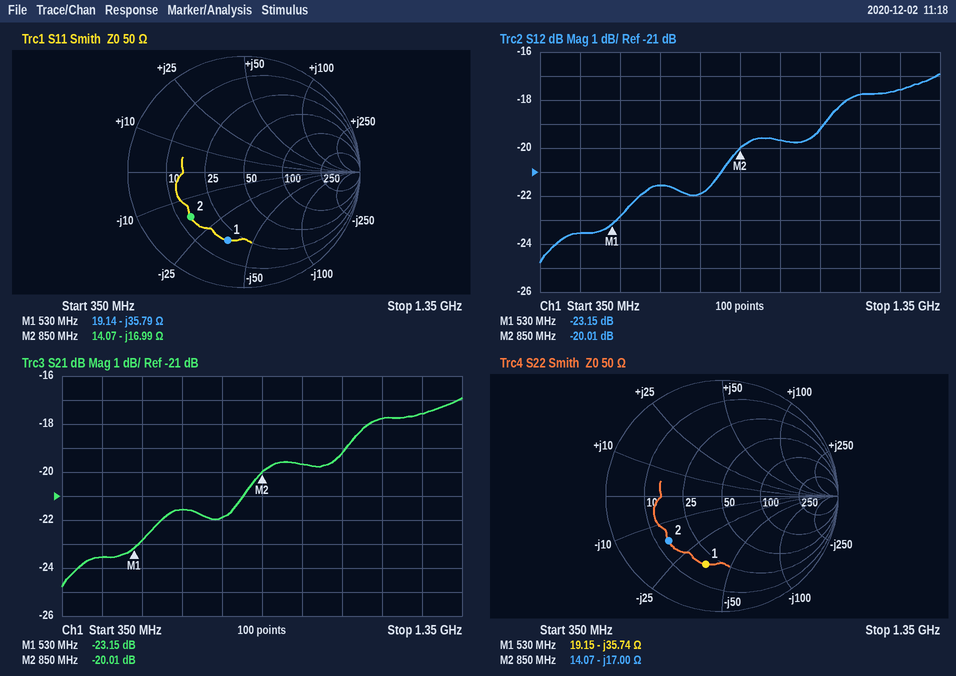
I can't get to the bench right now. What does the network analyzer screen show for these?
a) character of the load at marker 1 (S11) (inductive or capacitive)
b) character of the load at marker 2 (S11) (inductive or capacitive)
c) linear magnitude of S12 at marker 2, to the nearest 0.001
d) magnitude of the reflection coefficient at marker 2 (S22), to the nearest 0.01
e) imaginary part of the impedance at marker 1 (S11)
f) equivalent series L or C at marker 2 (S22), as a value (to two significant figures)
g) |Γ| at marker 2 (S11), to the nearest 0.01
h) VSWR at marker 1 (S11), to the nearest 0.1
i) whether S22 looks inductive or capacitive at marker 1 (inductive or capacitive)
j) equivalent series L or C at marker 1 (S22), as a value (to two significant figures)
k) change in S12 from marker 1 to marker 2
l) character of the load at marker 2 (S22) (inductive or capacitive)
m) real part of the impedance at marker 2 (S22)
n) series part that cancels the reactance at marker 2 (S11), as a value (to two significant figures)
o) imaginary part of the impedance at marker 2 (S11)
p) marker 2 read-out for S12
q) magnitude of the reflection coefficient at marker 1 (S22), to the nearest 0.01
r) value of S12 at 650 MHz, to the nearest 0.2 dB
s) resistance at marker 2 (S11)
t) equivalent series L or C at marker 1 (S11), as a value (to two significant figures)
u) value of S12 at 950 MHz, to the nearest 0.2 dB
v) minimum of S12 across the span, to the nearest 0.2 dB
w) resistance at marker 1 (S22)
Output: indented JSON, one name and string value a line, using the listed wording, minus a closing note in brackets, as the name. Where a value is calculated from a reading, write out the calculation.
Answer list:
{
  "character of the load at marker 1 (S11)": "capacitive",
  "character of the load at marker 2 (S11)": "capacitive",
  "linear magnitude of S12 at marker 2, to the nearest 0.001": "10^(-20.01/20) ≈ 0.100",
  "magnitude of the reflection coefficient at marker 2 (S22), to the nearest 0.01": "0.60",
  "imaginary part of the impedance at marker 1": "-35.79 Ω",
  "equivalent series L or C at marker 2 (S22), as a value": "C = 1/(2π × 850 MHz × 17 Ω) ≈ 11 pF",
  "|Γ| at marker 2 (S11), to the nearest 0.01": "0.60",
  "VSWR at marker 1 (S11), to the nearest 0.1": "4.1",
  "whether S22 looks inductive or capacitive at marker 1": "capacitive",
  "equivalent series L or C at marker 1 (S22), as a value": "C = 1/(2π × 530 MHz × 35.74 Ω) ≈ 8.4 pF",
  "change in S12 from marker 1 to marker 2": "-20.01 − (-23.15) = 3.14 dB",
  "character of the load at marker 2 (S22)": "capacitive",
  "real part of the impedance at marker 2": "14.07 Ω",
  "series part that cancels the reactance at marker 2 (S11), as a value": "L = 16.99 Ω/(2π × 850 MHz) ≈ 3.2 nH",
  "imaginary part of the impedance at marker 2": "-16.99 Ω",
  "marker 2 read-out for S12": "-20.01 dB",
  "magnitude of the reflection coefficient at marker 1 (S22), to the nearest 0.01": "0.61",
  "value of S12 at 650 MHz, to the nearest 0.2 dB": "-21.6 dB",
  "resistance at marker 2": "14.07 Ω",
  "equivalent series L or C at marker 1 (S11), as a value": "C = 1/(2π × 530 MHz × 35.79 Ω) ≈ 8.4 pF",
  "value of S12 at 950 MHz, to the nearest 0.2 dB": "-19.6 dB",
  "minimum of S12 across the span, to the nearest 0.2 dB": "-24.8 dB",
  "resistance at marker 1": "19.15 Ω"
}
